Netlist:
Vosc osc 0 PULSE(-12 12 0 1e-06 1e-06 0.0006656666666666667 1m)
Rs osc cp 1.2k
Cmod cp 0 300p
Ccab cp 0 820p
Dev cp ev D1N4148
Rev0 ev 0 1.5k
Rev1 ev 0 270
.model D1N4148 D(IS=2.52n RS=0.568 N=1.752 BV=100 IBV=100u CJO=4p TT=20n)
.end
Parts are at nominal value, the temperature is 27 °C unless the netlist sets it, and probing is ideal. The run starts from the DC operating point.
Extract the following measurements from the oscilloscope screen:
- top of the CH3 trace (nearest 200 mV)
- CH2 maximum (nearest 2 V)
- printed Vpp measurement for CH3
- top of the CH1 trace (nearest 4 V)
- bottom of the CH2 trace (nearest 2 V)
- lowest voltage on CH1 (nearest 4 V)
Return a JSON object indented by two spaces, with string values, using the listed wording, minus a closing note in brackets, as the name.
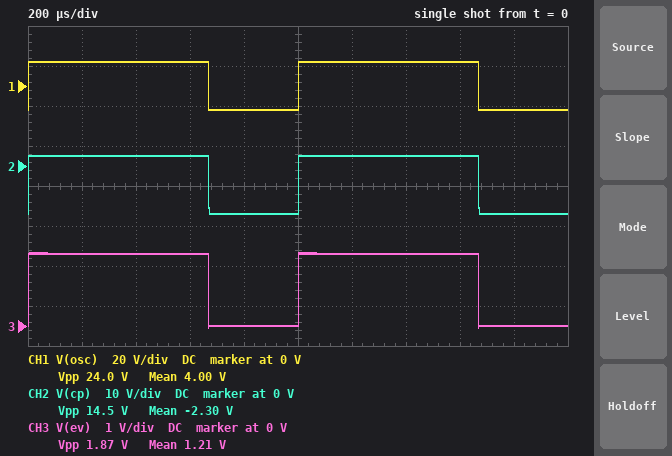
{
  "top of the CH3 trace": "1.8 V",
  "CH2 maximum": "2 V",
  "printed Vpp measurement for CH3": "1.87 V",
  "top of the CH1 trace": "12 V",
  "bottom of the CH2 trace": "-12 V",
  "lowest voltage on CH1": "-12 V"
}
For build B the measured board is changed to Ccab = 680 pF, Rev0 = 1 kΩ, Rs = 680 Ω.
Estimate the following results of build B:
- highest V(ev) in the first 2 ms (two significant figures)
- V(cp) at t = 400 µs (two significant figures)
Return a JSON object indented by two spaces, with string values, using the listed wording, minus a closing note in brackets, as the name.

{
  "highest V(ev) in the first 2 ms": "2.7 V",
  "V(cp) at t = 400 µs": "3.4 V"
}
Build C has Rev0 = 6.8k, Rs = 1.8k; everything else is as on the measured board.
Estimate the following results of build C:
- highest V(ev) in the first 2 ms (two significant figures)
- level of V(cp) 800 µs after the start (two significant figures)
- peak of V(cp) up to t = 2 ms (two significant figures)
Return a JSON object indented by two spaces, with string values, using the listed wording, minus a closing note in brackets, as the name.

{
  "highest V(ev) in the first 2 ms": "1.4 V",
  "level of V(cp) 800 µs after the start": "-12 V",
  "peak of V(cp) up to t = 2 ms": "2.1 V"
}
